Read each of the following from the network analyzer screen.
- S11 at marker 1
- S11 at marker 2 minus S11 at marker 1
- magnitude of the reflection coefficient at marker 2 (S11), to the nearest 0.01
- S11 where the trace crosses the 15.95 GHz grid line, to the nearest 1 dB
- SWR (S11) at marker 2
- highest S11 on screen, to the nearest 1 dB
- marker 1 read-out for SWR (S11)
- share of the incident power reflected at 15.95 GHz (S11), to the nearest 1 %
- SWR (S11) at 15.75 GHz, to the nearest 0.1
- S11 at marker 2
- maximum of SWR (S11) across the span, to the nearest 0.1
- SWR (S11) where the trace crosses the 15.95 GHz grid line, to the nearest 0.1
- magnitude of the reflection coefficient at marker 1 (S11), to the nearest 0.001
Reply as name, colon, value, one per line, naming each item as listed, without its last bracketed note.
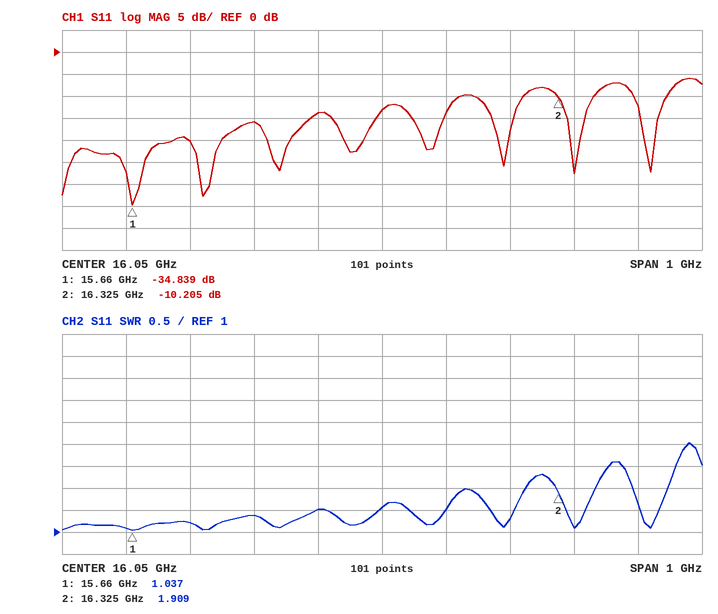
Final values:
S11 at marker 1: -34.839 dB
S11 at marker 2 minus S11 at marker 1: 24.634 dB
magnitude of the reflection coefficient at marker 2 (S11), to the nearest 0.01: 0.31
S11 where the trace crosses the 15.95 GHz grid line, to the nearest 1 dB: -14 dB
SWR (S11) at marker 2: 1.909
highest S11 on screen, to the nearest 1 dB: -6 dB
marker 1 read-out for SWR: 1.037
share of the incident power reflected at 15.95 GHz (S11), to the nearest 1 %: 4 %
SWR (S11) at 15.75 GHz, to the nearest 0.1: 1.2
S11 at marker 2: -10.205 dB
maximum of SWR (S11) across the span, to the nearest 0.1: 3.0
SWR (S11) where the trace crosses the 15.95 GHz grid line, to the nearest 0.1: 1.5
magnitude of the reflection coefficient at marker 1 (S11), to the nearest 0.001: 0.018
